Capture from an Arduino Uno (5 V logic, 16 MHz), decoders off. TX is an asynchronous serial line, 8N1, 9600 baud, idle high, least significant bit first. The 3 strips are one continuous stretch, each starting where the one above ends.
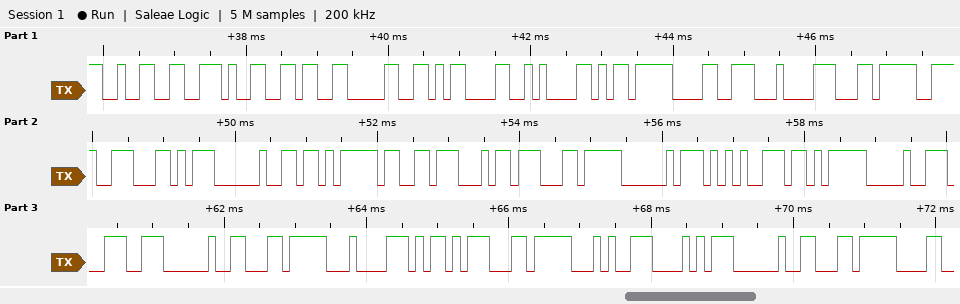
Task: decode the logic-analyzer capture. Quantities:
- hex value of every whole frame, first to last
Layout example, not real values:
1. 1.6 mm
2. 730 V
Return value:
1. 32 2E 36 30 0D 0A ED 98 84 EC 9E AC 20 EB B3 B4 EC A0 95 EB 90 9C 20 EC 84 AD EC 94 A8 20 EC
